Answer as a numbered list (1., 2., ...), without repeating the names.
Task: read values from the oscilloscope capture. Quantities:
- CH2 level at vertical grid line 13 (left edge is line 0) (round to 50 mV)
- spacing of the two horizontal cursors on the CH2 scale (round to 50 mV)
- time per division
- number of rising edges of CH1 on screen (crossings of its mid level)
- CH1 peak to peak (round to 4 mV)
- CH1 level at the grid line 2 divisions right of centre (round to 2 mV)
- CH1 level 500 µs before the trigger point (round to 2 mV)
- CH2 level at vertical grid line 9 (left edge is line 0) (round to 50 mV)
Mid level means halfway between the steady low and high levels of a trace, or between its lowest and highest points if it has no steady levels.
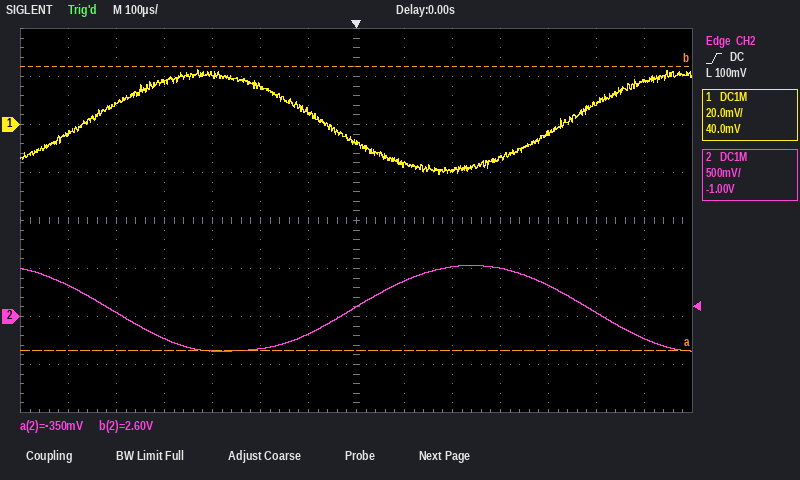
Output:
1. -250 mV
2. 2.95 V
3. 100 µs
4. 2
5. 44 mV
6. -20 mV
7. 8 mV
8. 500 mV
